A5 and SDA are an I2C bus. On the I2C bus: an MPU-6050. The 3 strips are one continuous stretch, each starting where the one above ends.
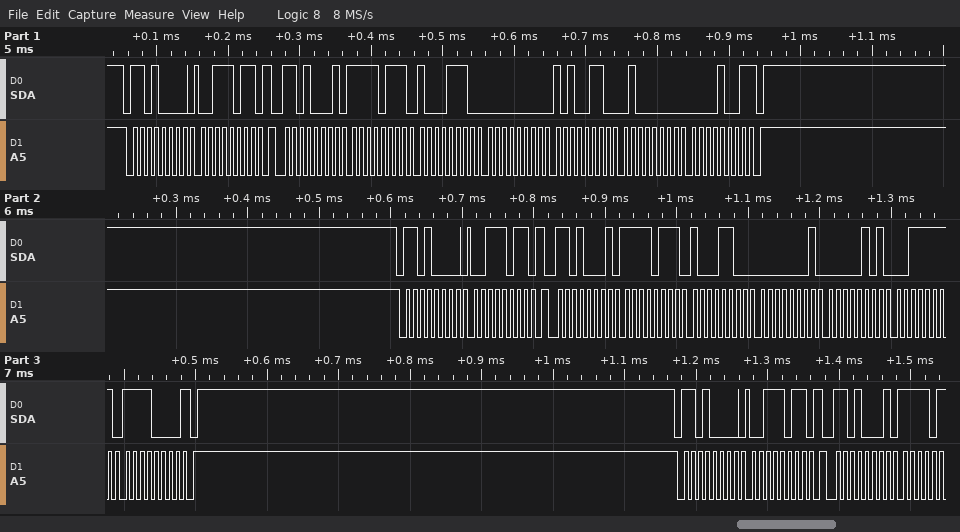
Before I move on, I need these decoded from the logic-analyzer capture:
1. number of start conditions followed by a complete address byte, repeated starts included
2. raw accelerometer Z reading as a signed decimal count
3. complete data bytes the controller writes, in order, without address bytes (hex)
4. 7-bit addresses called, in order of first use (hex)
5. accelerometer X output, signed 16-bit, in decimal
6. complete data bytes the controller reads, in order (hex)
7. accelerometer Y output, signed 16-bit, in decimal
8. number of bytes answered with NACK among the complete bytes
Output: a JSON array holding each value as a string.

["6", "16393", "3B 3B 3B", "0x68", "-2162", "F7 8E 00 A6 40 09 F7 8C 01 05 3F F0", "166", "2"]
